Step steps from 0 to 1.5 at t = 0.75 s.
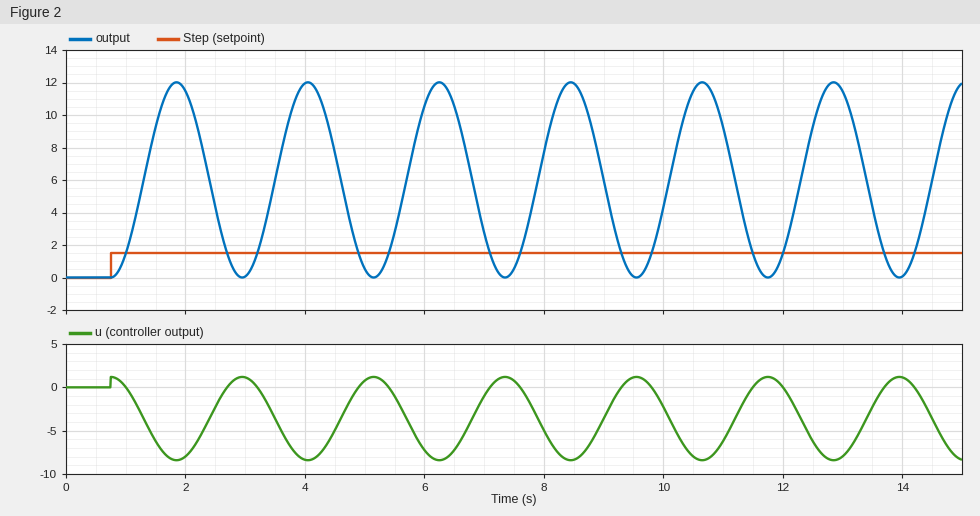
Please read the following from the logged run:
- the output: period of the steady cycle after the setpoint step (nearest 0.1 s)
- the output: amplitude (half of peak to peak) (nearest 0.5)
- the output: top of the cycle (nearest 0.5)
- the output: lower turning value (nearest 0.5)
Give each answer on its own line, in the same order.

2.2 s
6.0
12.0
0.0
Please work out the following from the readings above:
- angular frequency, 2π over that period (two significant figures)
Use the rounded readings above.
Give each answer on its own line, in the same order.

2.9 rad/s
